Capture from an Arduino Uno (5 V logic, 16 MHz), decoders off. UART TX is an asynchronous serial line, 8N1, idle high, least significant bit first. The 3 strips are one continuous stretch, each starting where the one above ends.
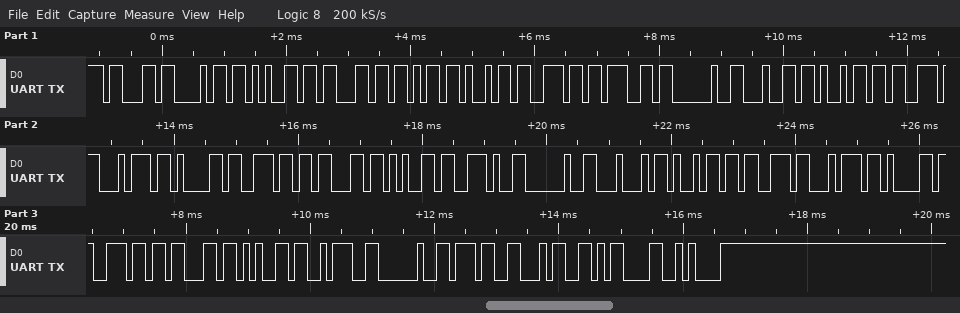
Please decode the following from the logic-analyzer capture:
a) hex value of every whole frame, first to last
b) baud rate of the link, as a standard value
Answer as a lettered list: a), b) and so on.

a) 63 68 65 63 6B 69 6E 67 20 64 69 73 74 61 6E 63 65 2E 20 44 69 73 74 61 6E 63 65 3A 20 37 34 0D 0A
b) 9600 baud
